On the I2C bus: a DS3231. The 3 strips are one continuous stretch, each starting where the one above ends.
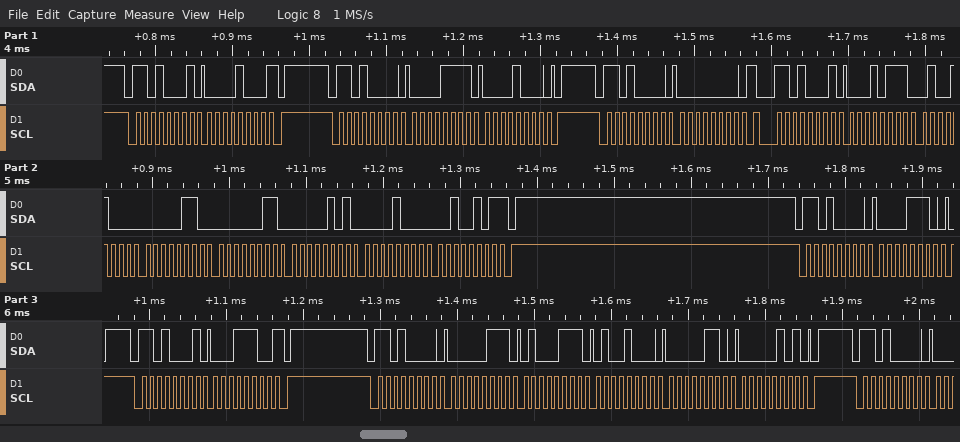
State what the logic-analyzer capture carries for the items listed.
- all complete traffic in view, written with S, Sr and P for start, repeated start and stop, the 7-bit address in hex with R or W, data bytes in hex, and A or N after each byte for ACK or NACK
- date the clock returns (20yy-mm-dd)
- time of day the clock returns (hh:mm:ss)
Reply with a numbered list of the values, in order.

1. S 68R A 08 N P S 68W A 0F A 08 A P S 68W A 00 A Sr 68R A 17 A 48 A 06 A 03 A 05 A 08 A 25 N P S 68W A 0E A P S 68R A 1C N P S 68W A 07 A 47 A 48 A 06 A 05 A P S 68W A
2. 2025-08-05
3. 06:48:17
